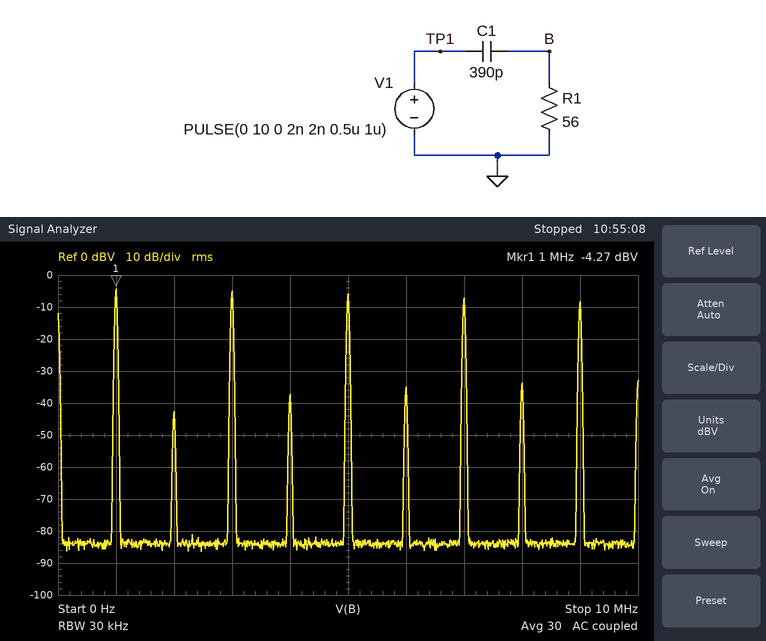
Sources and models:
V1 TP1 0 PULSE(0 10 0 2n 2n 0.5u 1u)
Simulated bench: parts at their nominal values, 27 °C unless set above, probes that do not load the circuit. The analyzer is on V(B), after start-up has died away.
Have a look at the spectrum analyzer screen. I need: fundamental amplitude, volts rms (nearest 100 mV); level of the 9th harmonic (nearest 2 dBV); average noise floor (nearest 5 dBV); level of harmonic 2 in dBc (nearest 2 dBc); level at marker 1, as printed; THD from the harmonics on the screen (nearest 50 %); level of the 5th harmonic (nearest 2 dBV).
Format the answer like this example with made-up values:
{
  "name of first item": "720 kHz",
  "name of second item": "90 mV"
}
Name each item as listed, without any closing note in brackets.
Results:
{
  "fundamental amplitude, volts rms": "600 mV",
  "level of the 9th harmonic": "-8 dBV",
  "average noise floor": "-85 dBV",
  "level of harmonic 2 in dBc": "-38 dBc",
  "level at marker 1, as printed": "-4.27 dBV",
  "THD from the harmonics on the screen": "150 %",
  "level of the 5th harmonic": "-6 dBV"
}
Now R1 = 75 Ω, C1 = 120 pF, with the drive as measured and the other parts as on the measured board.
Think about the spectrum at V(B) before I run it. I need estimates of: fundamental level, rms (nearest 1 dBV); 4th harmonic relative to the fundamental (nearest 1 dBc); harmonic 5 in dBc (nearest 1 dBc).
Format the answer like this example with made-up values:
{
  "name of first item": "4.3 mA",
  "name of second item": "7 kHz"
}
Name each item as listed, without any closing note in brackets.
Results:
{
  "fundamental level, rms": "-12 dBV",
  "4th harmonic relative to the fundamental": "-32 dBc",
  "harmonic 5 in dBc": "0 dBc"
}
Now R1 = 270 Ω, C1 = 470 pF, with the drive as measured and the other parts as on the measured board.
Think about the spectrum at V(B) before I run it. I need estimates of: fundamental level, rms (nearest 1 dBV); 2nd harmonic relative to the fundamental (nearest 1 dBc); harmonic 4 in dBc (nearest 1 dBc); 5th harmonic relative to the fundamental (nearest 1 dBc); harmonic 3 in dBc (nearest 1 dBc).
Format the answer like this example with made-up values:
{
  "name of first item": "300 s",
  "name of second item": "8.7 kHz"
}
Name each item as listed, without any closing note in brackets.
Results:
{
  "fundamental level, rms": "9 dBV",
  "2nd harmonic relative to the fundamental": "-41 dBc",
  "harmonic 4 in dBc": "-40 dBc",
  "5th harmonic relative to the fundamental": "-10 dBc",
  "harmonic 3 in dBc": "-6 dBc"
}
